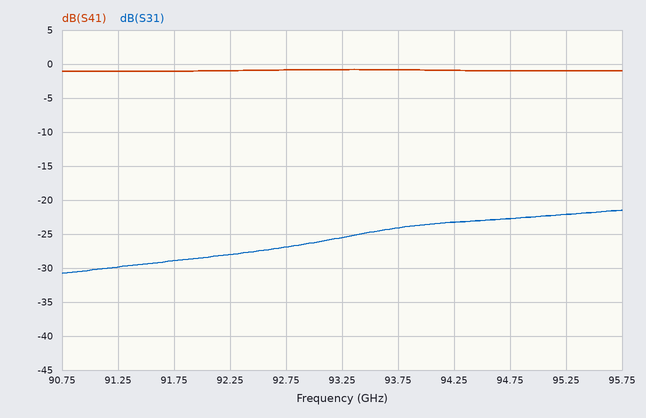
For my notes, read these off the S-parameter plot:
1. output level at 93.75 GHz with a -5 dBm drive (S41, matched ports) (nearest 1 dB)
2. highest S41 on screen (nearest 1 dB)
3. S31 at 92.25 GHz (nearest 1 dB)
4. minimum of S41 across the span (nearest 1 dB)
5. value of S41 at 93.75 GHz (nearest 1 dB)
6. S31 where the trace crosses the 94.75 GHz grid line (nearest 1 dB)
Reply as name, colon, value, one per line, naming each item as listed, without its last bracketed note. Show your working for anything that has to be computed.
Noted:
output level at 93.75 GHz with a -5 dBm drive (S41, matched ports): -5 dBm + (-1 dB) = -6 dBm
highest S41 on screen: -1 dB
S31 at 92.25 GHz: -28 dB
minimum of S41 across the span: -1 dB
value of S41 at 93.75 GHz: -1 dB
S31 where the trace crosses the 94.75 GHz grid line: -23 dB
